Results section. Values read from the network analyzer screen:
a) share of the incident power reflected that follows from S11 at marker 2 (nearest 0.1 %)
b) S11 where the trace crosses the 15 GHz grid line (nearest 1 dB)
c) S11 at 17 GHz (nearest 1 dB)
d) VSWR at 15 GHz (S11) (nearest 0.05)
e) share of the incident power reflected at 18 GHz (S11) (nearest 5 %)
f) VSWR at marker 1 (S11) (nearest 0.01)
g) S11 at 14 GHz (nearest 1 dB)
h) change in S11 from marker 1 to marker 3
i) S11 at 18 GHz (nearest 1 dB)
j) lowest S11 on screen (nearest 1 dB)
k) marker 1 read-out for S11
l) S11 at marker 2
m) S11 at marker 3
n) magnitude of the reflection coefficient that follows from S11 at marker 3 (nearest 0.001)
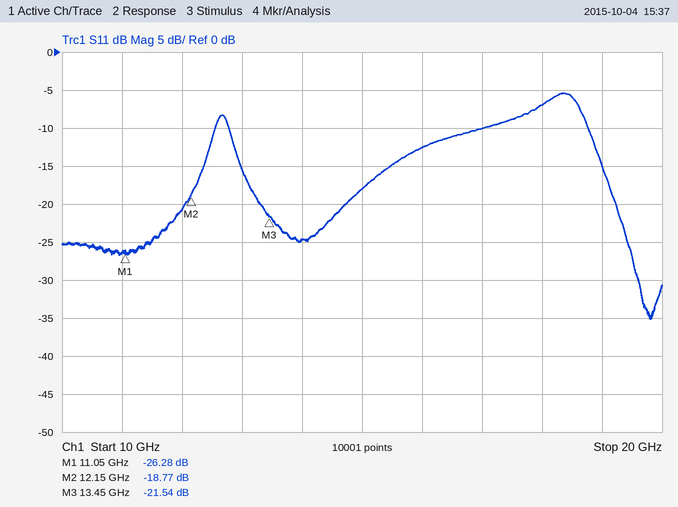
1.3 %
-18 dB
-10 dB
1.30
20 %
1.10
-25 dB
4.74 dB
-7 dB
-35 dB
-26.28 dB
-18.77 dB
-21.54 dB
0.084
